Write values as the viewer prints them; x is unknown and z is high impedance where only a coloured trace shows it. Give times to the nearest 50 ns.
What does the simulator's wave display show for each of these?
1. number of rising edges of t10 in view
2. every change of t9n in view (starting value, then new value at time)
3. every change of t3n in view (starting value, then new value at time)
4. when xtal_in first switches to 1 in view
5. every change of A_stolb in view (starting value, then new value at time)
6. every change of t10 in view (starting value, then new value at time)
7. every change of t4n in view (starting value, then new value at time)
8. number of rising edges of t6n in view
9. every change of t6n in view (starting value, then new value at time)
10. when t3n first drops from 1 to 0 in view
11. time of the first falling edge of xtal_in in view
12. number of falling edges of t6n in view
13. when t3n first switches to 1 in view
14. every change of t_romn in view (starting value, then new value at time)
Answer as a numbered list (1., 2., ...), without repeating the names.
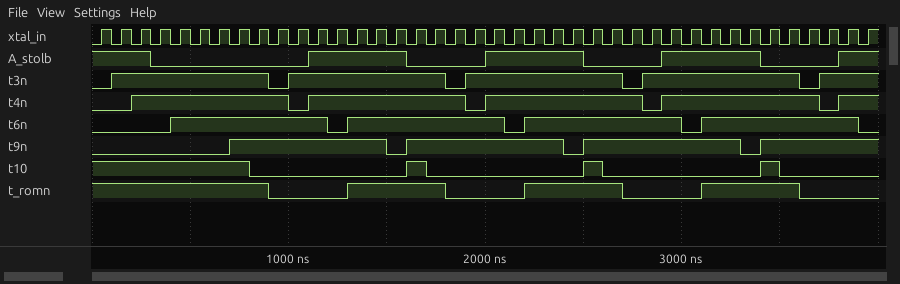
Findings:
1. 3
2. 0, 1 at 700 ns, 0 at 1500 ns, 1 at 1600 ns, 0 at 2400 ns, 1 at 2500 ns, 0 at 3300 ns, 1 at 3400 ns
3. 0, 1 at 100 ns, 0 at 900 ns, 1 at 1000 ns, 0 at 1800 ns, 1 at 1900 ns, 0 at 2700 ns, 1 at 2800 ns, 0 at 3600 ns, 1 at 3700 ns
4. 50 ns
5. 1, 0 at 300 ns, 1 at 1100 ns, 0 at 1600 ns, 1 at 2000 ns, 0 at 2500 ns, 1 at 2900 ns, 0 at 3400 ns, 1 at 3800 ns
6. 1, 0 at 800 ns, 1 at 1600 ns, 0 at 1700 ns, 1 at 2500 ns, 0 at 2600 ns, 1 at 3400 ns, 0 at 3500 ns
7. 0, 1 at 200 ns, 0 at 1000 ns, 1 at 1100 ns, 0 at 1900 ns, 1 at 2000 ns, 0 at 2800 ns, 1 at 2900 ns, 0 at 3700 ns, 1 at 3800 ns
8. 4
9. 0, 1 at 400 ns, 0 at 1200 ns, 1 at 1300 ns, 0 at 2100 ns, 1 at 2200 ns, 0 at 3000 ns, 1 at 3100 ns, 0 at 3900 ns
10. 900 ns
11. 100 ns
12. 4
13. 100 ns
14. 1, 0 at 900 ns, 1 at 1300 ns, 0 at 1800 ns, 1 at 2200 ns, 0 at 2700 ns, 1 at 3100 ns, 0 at 3600 ns
